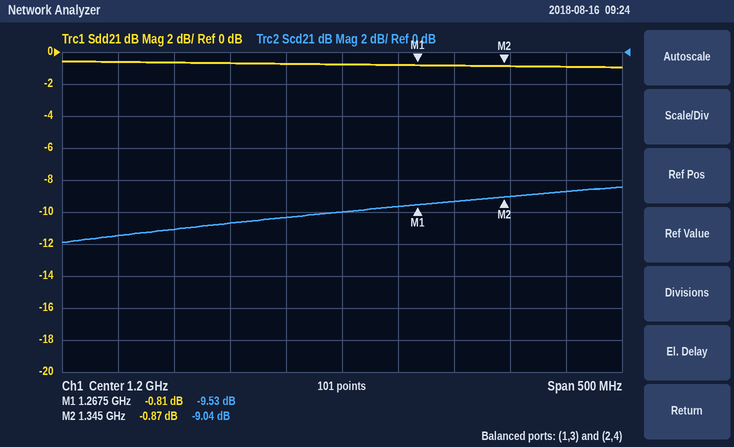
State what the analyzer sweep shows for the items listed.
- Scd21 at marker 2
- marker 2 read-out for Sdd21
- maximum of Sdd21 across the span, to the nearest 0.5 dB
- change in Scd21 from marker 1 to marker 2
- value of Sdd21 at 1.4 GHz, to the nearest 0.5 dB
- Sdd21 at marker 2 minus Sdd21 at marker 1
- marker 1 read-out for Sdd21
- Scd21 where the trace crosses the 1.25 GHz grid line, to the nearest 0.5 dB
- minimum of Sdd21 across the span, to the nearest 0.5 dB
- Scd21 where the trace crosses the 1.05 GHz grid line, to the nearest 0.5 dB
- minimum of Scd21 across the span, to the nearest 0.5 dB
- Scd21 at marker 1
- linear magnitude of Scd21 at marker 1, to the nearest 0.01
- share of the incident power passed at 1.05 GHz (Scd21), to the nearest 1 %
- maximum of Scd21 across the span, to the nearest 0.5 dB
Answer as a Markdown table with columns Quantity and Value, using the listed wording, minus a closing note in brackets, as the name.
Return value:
| Quantity | Value |
|---|---|
| Scd21 at marker 2 | -9.04 dB |
| marker 2 read-out for Sdd21 | -0.87 dB |
| maximum of Sdd21 across the span, to the nearest 0.5 dB | -0.5 dB |
| change in Scd21 from marker 1 to marker 2 | 0.49 dB |
| value of Sdd21 at 1.4 GHz, to the nearest 0.5 dB | -1.0 dB |
| Sdd21 at marker 2 minus Sdd21 at marker 1 | -0.06 dB |
| marker 1 read-out for Sdd21 | -0.81 dB |
| Scd21 where the trace crosses the 1.25 GHz grid line, to the nearest 0.5 dB | -9.5 dB |
| minimum of Sdd21 across the span, to the nearest 0.5 dB | -1.0 dB |
| Scd21 where the trace crosses the 1.05 GHz grid line, to the nearest 0.5 dB | -11.0 dB |
| minimum of Scd21 across the span, to the nearest 0.5 dB | -12.0 dB |
| Scd21 at marker 1 | -9.53 dB |
| linear magnitude of Scd21 at marker 1, to the nearest 0.01 | 0.33 |
| share of the incident power passed at 1.05 GHz (Scd21), to the nearest 1 % | 8 % |
| maximum of Scd21 across the span, to the nearest 0.5 dB | -8.5 dB |
